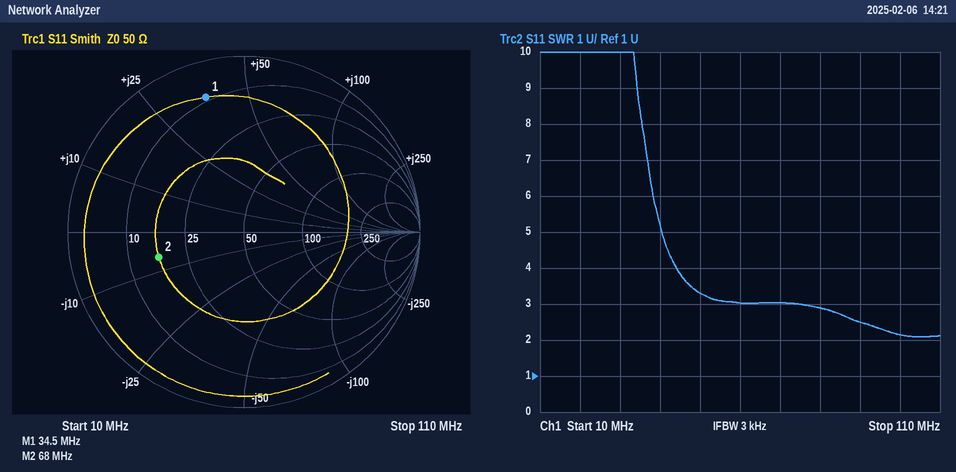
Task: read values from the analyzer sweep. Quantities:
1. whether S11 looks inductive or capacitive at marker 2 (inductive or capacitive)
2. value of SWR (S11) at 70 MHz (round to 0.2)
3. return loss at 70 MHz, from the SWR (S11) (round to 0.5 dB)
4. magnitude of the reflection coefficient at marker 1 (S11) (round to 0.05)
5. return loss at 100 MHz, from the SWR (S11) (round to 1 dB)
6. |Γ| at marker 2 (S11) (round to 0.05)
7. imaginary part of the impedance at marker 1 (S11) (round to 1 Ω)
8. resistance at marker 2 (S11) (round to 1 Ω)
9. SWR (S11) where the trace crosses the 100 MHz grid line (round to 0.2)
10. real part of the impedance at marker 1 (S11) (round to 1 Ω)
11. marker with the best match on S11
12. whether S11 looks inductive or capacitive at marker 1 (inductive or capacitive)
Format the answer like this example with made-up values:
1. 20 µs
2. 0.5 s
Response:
1. capacitive
2. 3.0
3. 6.0 dB
4. 0.80
5. 9 dB
6. 0.50
7. +37 Ω
8. 17 Ω
9. 2.2
10. 9 Ω
11. marker 2
12. inductive
